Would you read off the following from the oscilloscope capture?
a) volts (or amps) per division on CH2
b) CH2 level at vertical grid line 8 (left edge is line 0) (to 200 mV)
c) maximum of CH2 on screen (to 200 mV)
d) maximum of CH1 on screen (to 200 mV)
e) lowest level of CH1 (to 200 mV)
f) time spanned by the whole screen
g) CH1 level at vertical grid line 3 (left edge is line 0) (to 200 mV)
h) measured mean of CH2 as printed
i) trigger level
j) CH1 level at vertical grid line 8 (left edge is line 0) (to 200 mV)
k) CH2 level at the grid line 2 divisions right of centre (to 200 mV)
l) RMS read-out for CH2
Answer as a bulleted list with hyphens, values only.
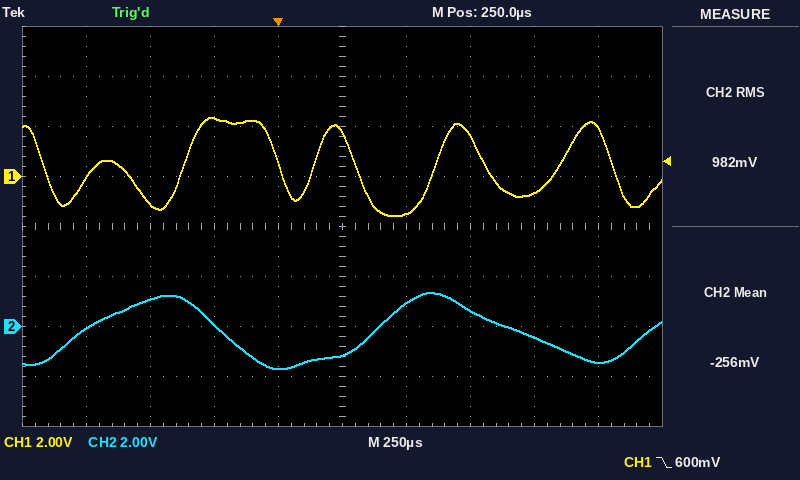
- 2 V
- -400 mV
- 1.4 V
- 2.4 V
- -1.6 V
- 2.5 ms
- 2.4 V
- -256 mV
- 600 mV
- -600 mV
- 600 mV
- 982 mV
